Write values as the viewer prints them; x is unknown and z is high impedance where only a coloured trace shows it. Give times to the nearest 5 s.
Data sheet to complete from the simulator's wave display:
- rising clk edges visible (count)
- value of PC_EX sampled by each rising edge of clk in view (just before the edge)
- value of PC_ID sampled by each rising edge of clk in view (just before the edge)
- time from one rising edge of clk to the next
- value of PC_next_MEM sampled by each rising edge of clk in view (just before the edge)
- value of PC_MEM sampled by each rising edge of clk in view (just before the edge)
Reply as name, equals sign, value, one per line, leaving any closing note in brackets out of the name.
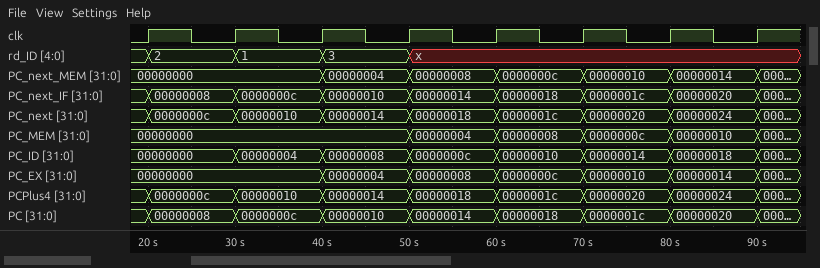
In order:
rising clk edges visible = 8
value of PC_EX sampled by each rising edge of clk in view = 00000000, 00000000, 00000000, 00000004, 00000008, 0000000c, 00000010, 00000014
value of PC_ID sampled by each rising edge of clk in view = 00000000, 00000000, 00000004, 00000008, 0000000c, 00000010, 00000014, 00000018
time from one rising edge of clk to the next = 10 s
value of PC_next_MEM sampled by each rising edge of clk in view = 00000000, 00000000, 00000000, 00000004, 00000008, 0000000c, 00000010, 00000014
value of PC_MEM sampled by each rising edge of clk in view = 00000000, 00000000, 00000000, 00000000, 00000004, 00000008, 0000000c, 00000010
